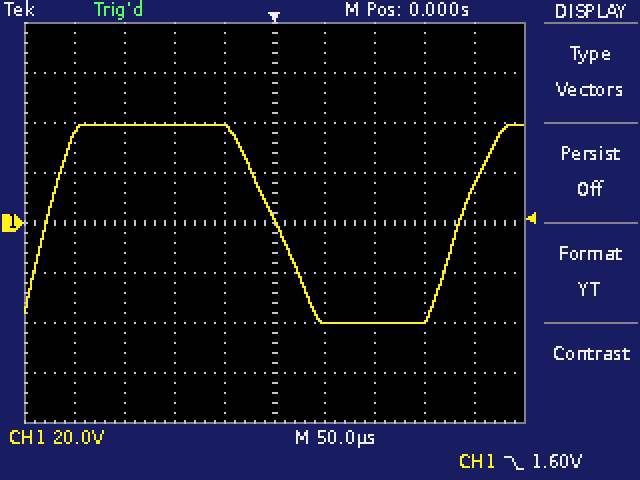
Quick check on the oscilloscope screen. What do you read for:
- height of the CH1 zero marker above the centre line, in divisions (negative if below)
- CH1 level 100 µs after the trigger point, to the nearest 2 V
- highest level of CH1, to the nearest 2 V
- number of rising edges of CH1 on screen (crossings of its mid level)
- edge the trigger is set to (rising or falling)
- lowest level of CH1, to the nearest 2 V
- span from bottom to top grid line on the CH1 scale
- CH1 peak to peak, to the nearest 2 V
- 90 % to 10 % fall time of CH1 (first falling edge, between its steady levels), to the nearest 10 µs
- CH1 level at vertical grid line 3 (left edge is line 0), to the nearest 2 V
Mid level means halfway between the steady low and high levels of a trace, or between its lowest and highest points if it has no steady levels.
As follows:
0.0 div
-40 V
40 V
2
falling
-40 V
160 V
80 V
70 µs
40 V
